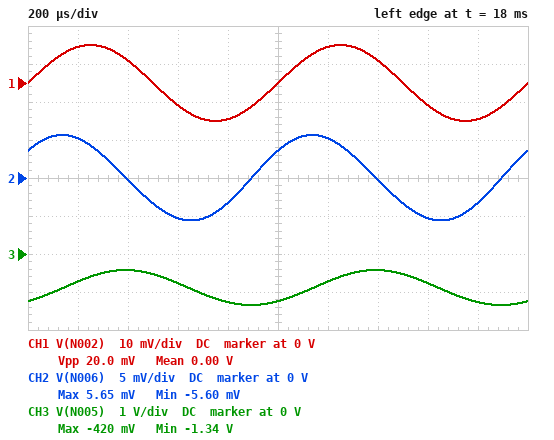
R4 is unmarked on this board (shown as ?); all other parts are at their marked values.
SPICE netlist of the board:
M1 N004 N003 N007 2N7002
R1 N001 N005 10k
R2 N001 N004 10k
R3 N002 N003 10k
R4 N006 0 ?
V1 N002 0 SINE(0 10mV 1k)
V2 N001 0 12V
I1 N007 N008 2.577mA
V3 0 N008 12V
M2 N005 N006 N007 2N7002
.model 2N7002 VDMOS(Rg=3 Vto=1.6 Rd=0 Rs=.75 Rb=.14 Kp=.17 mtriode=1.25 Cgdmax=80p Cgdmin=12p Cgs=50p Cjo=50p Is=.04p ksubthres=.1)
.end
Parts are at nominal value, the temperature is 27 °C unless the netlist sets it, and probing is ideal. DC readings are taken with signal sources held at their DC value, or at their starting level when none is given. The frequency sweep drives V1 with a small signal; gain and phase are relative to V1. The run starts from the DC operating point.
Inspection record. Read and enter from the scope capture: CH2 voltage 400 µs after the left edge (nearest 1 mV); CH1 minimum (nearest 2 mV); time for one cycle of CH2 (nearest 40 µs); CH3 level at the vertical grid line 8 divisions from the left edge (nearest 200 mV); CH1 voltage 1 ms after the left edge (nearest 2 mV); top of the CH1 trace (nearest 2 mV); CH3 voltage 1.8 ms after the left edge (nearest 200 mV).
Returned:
0 V
-10 mV
1.00 ms
-800 mV
0 V
10 mV
-1.2 V
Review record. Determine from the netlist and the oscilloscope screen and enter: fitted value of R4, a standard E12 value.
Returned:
27 kΩ
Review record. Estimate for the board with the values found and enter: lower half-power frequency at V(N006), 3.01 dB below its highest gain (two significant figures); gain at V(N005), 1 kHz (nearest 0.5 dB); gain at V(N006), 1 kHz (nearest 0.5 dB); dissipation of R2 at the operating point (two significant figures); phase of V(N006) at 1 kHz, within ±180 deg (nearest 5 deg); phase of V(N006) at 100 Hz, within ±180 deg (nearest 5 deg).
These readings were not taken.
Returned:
780 Hz
33.0 dB
-5.0 dB
17 mW
40 deg
85 deg
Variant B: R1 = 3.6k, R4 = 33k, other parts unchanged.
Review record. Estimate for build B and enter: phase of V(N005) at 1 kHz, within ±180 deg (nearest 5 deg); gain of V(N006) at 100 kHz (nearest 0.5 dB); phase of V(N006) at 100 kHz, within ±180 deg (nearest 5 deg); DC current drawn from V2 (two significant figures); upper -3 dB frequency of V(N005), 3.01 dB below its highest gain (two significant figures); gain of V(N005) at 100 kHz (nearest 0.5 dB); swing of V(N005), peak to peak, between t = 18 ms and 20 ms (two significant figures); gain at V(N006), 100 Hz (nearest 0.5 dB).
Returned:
-25 deg
-13.5 dB
0 deg
2.6 mA
2.3 kHz
-4.0 dB
490 mV
-41.0 dB
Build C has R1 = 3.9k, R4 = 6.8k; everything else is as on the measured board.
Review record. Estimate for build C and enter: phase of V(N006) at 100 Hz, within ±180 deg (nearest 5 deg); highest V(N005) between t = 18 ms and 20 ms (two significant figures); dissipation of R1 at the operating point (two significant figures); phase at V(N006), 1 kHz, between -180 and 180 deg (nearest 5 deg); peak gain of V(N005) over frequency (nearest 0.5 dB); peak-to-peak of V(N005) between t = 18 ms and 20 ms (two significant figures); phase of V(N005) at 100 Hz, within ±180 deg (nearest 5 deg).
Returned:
90 deg
7.2 V
6.5 mW
70 deg
29.0 dB
540 mV
0 deg
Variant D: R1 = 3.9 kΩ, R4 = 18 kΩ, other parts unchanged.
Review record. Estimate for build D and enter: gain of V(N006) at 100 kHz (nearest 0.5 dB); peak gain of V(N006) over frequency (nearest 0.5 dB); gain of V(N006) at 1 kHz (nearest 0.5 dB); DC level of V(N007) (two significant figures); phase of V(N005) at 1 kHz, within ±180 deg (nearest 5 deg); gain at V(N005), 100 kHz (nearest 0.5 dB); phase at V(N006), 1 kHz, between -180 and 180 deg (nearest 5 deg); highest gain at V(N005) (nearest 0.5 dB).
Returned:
-17.0 dB
-14.0 dB
-26.0 dB
-1.7 V
-20 deg
-2.5 dB
70 deg
29.0 dB
